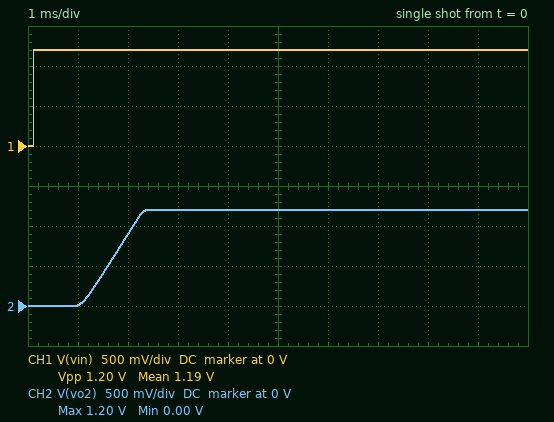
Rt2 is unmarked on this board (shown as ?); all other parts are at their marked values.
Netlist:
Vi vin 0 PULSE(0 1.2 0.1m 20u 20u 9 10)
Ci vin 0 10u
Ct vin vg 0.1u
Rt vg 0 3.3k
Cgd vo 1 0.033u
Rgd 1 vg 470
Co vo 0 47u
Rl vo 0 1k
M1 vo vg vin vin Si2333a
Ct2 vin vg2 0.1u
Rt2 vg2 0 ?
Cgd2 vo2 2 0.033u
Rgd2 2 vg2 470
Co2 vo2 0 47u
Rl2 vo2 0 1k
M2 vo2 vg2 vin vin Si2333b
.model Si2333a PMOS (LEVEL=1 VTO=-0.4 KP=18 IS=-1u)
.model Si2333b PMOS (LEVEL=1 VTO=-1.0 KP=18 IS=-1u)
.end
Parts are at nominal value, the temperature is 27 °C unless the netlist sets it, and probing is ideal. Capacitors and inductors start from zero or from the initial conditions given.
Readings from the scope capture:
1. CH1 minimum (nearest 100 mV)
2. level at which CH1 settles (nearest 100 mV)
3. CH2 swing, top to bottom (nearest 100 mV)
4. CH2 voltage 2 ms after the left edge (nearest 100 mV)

0 V
1.2 V
1.2 V
900 mV
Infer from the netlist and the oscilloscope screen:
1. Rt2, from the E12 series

3.9 kΩ
